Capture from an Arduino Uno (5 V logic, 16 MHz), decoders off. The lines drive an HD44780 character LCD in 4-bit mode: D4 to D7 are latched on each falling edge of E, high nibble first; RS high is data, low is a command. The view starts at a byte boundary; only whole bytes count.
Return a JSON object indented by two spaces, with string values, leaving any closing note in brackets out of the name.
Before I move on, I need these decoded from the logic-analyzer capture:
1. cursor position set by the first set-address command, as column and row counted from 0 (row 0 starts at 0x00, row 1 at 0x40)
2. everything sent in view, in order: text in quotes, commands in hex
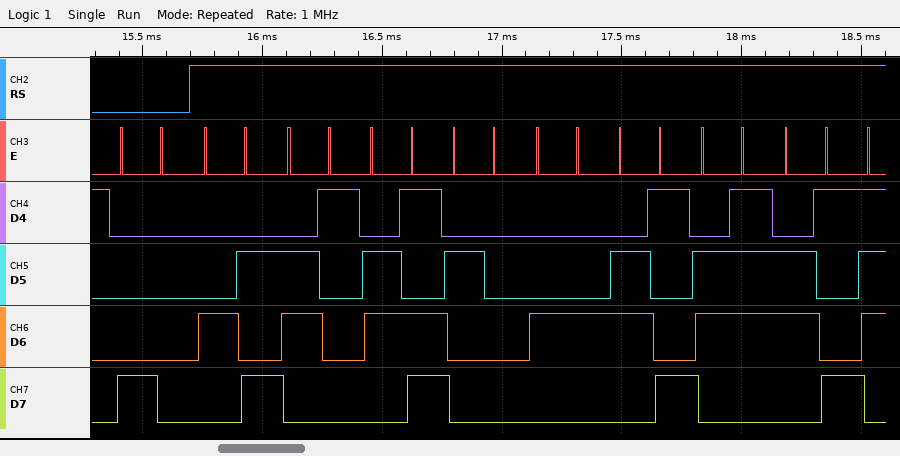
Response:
{
  "cursor position set by the first set-address command, as column and row counted from 0": "column 0, row 0",
  "everything sent in view, in order: text in quotes, commands in hex": "0x80 \"Jam Digi\""
}
